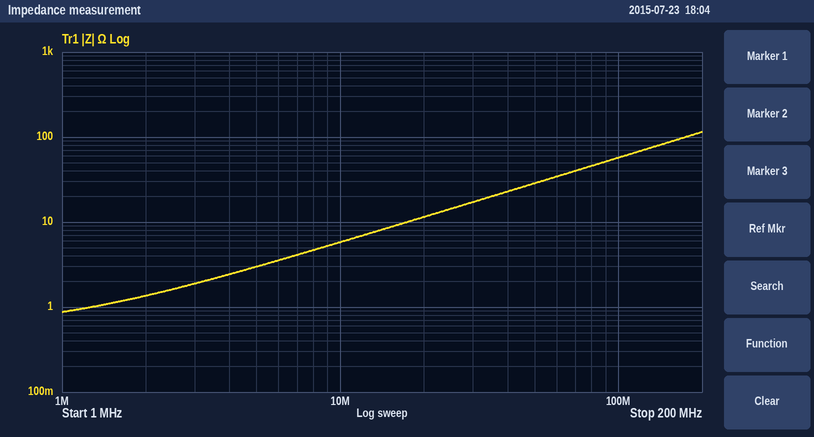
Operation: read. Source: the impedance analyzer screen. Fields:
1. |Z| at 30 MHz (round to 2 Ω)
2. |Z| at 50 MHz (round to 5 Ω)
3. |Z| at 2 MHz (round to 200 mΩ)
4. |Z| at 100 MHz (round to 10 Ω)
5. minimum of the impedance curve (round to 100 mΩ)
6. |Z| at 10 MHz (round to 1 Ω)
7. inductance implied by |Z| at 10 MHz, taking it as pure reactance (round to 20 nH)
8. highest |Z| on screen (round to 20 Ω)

18 Ω
30 Ω
1.4 Ω
60 Ω
900 mΩ
6 Ω
100 nH
120 Ω
